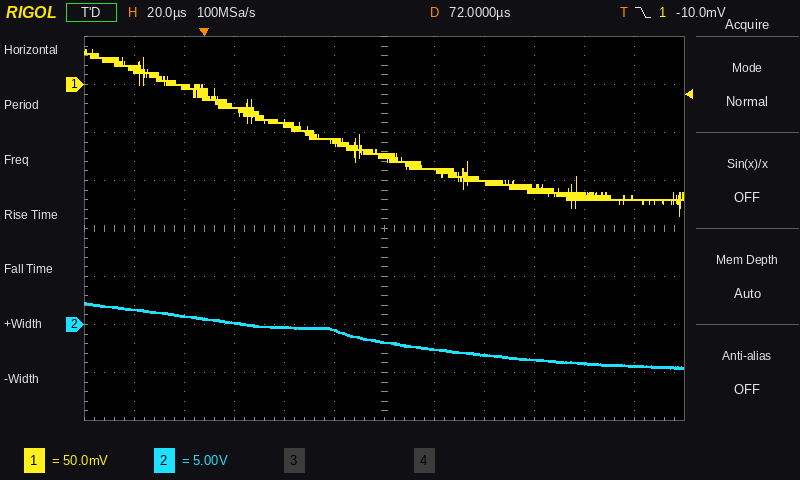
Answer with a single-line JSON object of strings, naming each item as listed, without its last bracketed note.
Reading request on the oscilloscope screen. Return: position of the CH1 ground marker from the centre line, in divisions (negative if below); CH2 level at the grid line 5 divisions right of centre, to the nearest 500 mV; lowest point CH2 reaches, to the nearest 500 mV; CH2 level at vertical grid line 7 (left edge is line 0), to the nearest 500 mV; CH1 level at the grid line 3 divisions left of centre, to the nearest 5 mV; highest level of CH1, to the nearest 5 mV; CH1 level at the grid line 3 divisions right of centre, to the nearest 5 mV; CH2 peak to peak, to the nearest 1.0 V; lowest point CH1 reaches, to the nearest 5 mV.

{"position of the CH1 ground marker from the centre line, in divisions": "+3.0 div", "CH2 level at the grid line 5 divisions right of centre, to the nearest 500 mV": "-4.5 V", "lowest point CH2 reaches, to the nearest 500 mV": "-4.5 V", "CH2 level at vertical grid line 7 (left edge is line 0), to the nearest 500 mV": "-2.5 V", "CH1 level at the grid line 3 divisions left of centre, to the nearest 5 mV": "-20 mV", "highest level of CH1, to the nearest 5 mV": "35 mV", "CH1 level at the grid line 3 divisions right of centre, to the nearest 5 mV": "-110 mV", "CH2 peak to peak, to the nearest 1.0 V": "7.0 V", "lowest point CH1 reaches, to the nearest 5 mV": "-135 mV"}
